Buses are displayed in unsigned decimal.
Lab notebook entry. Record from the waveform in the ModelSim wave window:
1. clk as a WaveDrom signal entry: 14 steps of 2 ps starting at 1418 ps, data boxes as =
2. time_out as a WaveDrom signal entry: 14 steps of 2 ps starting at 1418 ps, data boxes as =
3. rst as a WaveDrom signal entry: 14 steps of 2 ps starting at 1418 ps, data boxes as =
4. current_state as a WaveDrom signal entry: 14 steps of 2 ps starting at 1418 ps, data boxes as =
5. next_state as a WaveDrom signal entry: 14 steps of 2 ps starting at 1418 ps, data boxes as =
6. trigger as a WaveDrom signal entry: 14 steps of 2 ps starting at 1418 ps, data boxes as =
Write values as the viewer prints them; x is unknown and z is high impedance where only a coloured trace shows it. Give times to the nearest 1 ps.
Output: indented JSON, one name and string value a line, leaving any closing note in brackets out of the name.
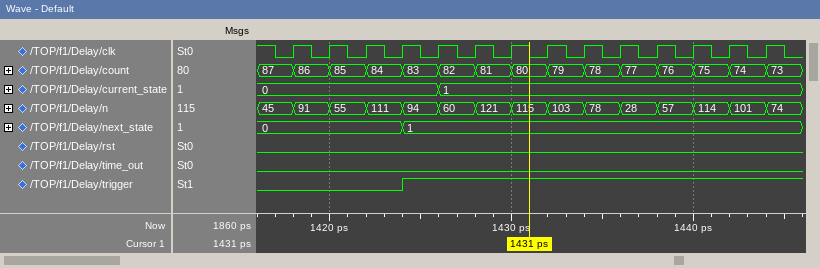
{
  "clk as a WaveDrom signal entry: 14 steps of 2 ps starting at 1418 ps, data boxes as =": "{name: 'clk', wave: 'p.............'}",
  "time_out as a WaveDrom signal entry: 14 steps of 2 ps starting at 1418 ps, data boxes as =": "{name: 'time_out', wave: '0.............'}",
  "rst as a WaveDrom signal entry: 14 steps of 2 ps starting at 1418 ps, data boxes as =": "{name: 'rst', wave: '0.............'}",
  "current_state as a WaveDrom signal entry: 14 steps of 2 ps starting at 1418 ps, data boxes as =": "{name: 'current_state', wave: '=...=.........', data: '0 1'}",
  "next_state as a WaveDrom signal entry: 14 steps of 2 ps starting at 1418 ps, data boxes as =": "{name: 'next_state', wave: '=..=..........', data: '0 1'}",
  "trigger as a WaveDrom signal entry: 14 steps of 2 ps starting at 1418 ps, data boxes as =": "{name: 'trigger', wave: '0..1..........'}"
}
